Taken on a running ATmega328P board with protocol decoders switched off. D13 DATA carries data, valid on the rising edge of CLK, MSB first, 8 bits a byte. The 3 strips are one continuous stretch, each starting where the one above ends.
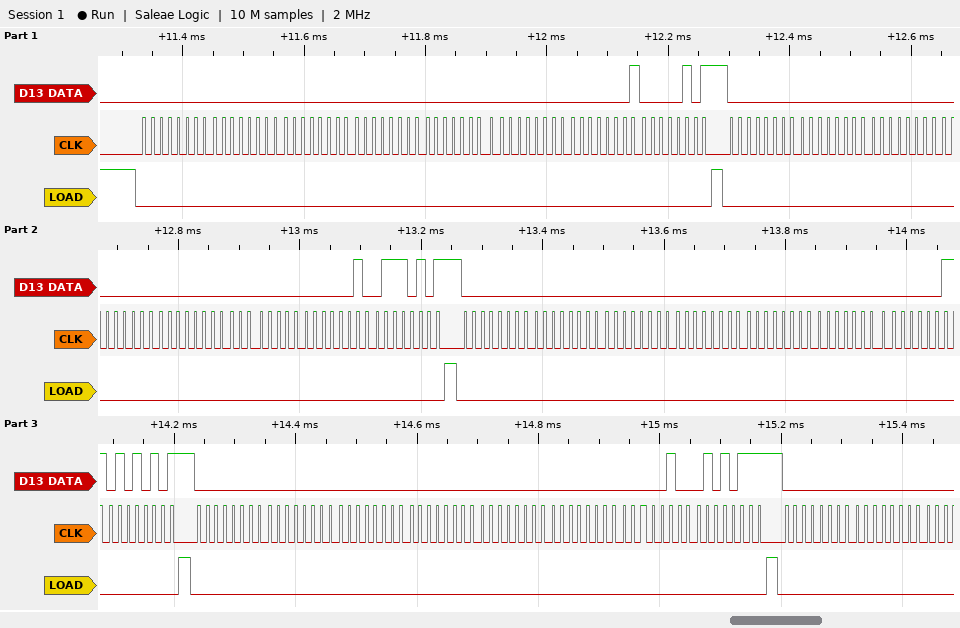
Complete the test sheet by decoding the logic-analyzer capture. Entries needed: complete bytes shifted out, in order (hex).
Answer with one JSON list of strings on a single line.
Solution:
["00 00 00 00 00 00 01 05 00 00 00 00 00 00 02 75 00 00 00 00 00 00 03 55 00 00 00 00 00 00 04 57 00 00"]
